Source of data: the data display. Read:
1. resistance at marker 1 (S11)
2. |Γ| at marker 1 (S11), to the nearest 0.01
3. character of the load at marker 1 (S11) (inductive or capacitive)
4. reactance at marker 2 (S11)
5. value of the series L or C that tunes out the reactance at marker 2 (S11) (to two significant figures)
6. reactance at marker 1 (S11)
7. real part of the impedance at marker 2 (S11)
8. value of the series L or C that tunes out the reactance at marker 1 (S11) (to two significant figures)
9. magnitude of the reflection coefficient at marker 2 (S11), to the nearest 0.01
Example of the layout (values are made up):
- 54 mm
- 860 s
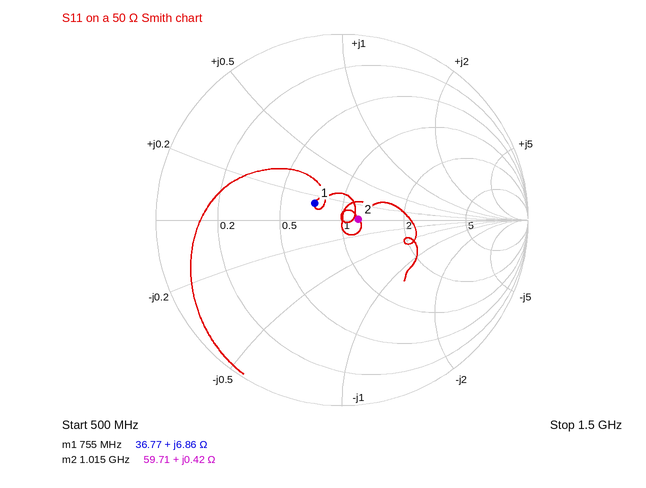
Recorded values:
- 36.77 Ω
- 0.17
- inductive
- +0.42 Ω
- 370 pF
- +6.86 Ω
- 59.71 Ω
- 31 pF
- 0.09
